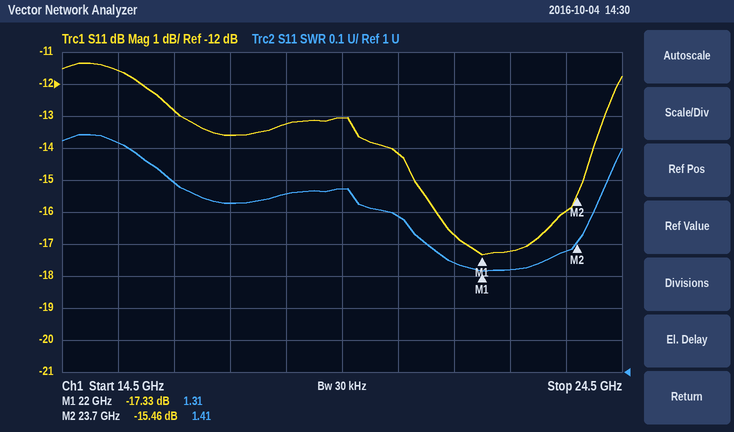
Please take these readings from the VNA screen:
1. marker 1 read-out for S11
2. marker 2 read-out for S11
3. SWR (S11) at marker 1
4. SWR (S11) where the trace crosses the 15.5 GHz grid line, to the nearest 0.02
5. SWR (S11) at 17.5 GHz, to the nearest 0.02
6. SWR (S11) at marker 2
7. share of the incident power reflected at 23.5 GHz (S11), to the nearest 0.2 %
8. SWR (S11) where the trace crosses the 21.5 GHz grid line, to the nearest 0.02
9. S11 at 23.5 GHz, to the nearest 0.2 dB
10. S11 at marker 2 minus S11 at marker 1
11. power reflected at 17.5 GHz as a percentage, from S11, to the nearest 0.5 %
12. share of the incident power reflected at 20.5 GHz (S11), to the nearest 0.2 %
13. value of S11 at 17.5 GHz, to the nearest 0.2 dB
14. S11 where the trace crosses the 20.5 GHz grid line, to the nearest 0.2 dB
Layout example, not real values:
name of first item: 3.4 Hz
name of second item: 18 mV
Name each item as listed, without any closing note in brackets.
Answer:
marker 1 read-out for S11: -17.33 dB
marker 2 read-out for S11: -15.46 dB
SWR (S11) at marker 1: 1.31
SWR (S11) where the trace crosses the 15.5 GHz grid line, to the nearest 0.02: 1.72
SWR (S11) at 17.5 GHz, to the nearest 0.02: 1.52
SWR (S11) at marker 2: 1.41
share of the incident power reflected at 23.5 GHz (S11), to the nearest 0.2 %: 2.6 %
SWR (S11) where the trace crosses the 21.5 GHz grid line, to the nearest 0.02: 1.34
S11 at 23.5 GHz, to the nearest 0.2 dB: -16.0 dB
S11 at marker 2 minus S11 at marker 1: 1.87 dB
power reflected at 17.5 GHz as a percentage, from S11, to the nearest 0.5 %: 4.5 %
share of the incident power reflected at 20.5 GHz (S11), to the nearest 0.2 %: 3.8 %
value of S11 at 17.5 GHz, to the nearest 0.2 dB: -13.6 dB
S11 where the trace crosses the 20.5 GHz grid line, to the nearest 0.2 dB: -14.2 dB
